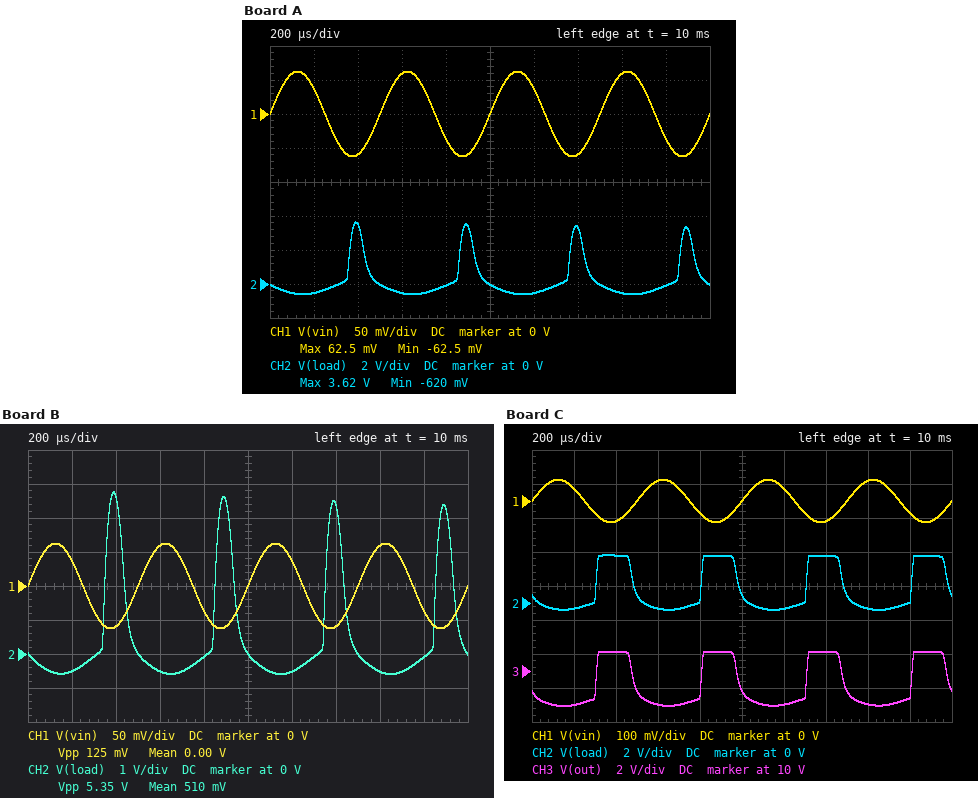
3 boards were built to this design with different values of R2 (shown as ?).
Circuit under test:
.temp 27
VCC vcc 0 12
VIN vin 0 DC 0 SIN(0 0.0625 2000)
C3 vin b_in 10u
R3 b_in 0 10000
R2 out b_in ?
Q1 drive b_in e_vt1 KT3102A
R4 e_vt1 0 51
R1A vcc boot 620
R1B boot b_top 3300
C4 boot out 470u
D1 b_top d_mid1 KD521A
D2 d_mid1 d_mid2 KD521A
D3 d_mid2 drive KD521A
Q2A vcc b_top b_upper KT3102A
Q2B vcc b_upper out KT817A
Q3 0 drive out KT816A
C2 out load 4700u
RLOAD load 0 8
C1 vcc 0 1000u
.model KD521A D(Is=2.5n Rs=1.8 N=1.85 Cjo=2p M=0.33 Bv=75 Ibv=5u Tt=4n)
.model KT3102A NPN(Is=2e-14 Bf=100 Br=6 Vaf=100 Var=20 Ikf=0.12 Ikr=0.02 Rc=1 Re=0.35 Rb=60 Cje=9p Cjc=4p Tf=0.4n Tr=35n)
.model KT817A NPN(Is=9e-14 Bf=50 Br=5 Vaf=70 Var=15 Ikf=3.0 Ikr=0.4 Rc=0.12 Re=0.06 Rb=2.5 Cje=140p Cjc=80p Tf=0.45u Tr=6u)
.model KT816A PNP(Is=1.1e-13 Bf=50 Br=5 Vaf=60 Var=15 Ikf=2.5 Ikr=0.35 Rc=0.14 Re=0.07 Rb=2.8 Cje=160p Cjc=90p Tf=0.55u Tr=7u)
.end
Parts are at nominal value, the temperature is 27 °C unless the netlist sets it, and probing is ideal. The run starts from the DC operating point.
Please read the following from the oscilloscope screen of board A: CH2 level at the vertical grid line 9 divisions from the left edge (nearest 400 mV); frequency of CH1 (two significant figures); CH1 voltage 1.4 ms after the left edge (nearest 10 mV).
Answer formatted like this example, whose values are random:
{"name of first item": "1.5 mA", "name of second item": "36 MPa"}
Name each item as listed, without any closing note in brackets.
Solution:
{"CH2 level at the vertical grid line 9 divisions from the left edge": "0 V", "frequency of CH1": "2.0 kHz", "CH1 voltage 1.4 ms after the left edge": "-60 mV"}
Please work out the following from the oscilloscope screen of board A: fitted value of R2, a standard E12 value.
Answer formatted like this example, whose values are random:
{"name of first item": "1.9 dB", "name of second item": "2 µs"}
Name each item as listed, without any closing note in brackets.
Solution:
{"fitted value of R2, a standard E12 value": "33 kΩ"}
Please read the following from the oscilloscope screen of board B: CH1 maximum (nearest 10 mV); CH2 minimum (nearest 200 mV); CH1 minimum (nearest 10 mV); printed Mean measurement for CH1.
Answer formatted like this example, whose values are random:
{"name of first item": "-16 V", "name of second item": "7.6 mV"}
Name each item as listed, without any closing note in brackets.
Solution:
{"CH1 maximum": "60 mV", "CH2 minimum": "-600 mV", "CH1 minimum": "-60 mV", "printed Mean measurement for CH1": "0.00 V"}
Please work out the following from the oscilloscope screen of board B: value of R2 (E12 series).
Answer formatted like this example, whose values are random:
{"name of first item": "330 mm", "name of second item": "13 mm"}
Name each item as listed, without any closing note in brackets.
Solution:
{"value of R2": "47 kΩ"}
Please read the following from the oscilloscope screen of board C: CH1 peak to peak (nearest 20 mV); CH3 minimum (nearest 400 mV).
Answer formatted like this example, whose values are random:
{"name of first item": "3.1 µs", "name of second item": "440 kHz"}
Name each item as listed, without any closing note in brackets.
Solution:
{"CH1 peak to peak": "120 mV", "CH3 minimum": "8.0 V"}
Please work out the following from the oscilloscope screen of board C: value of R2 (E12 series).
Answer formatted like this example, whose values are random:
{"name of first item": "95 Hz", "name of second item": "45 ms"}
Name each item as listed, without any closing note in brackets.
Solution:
{"value of R2": "100 kΩ"}
